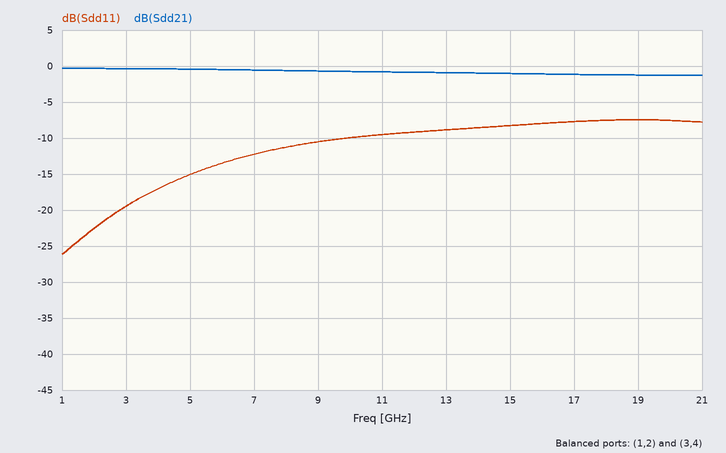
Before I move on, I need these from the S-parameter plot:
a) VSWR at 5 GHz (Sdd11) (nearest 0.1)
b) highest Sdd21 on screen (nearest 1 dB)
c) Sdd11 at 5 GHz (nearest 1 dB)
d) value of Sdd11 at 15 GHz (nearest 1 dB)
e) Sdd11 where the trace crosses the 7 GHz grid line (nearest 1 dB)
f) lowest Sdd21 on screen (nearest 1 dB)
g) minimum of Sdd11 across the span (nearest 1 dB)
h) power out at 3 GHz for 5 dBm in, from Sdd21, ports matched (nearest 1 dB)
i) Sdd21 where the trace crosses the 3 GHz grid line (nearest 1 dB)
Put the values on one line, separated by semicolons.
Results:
1.4; 0 dB; -15 dB; -8 dB; -12 dB; -1 dB; -26 dB; 5 dBm; 0 dB
